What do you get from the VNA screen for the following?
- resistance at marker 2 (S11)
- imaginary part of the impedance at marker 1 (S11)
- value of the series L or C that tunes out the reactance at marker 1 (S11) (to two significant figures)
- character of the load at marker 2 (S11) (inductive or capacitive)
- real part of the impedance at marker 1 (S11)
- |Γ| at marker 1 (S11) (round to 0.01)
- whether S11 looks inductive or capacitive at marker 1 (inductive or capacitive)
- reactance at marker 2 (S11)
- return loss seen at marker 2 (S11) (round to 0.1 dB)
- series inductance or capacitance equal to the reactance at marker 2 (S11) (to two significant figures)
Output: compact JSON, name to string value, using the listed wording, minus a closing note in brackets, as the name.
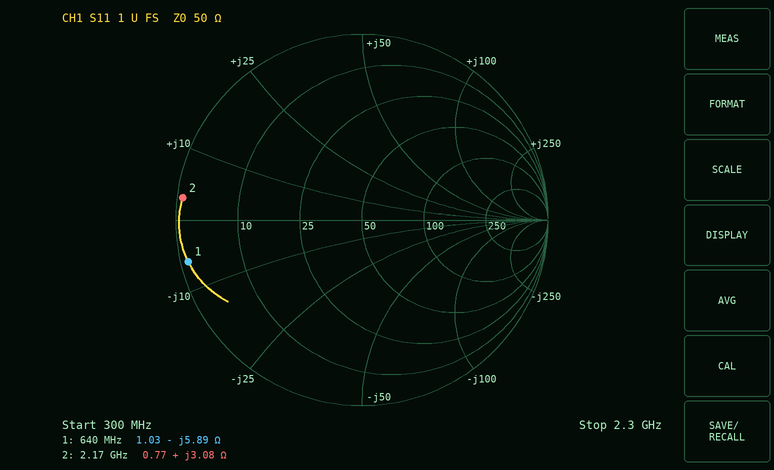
{"resistance at marker 2": "0.77 Ω", "imaginary part of the impedance at marker 1": "-5.89 Ω", "value of the series L or C that tunes out the reactance at marker 1 (S11)": "1.5 nH", "character of the load at marker 2 (S11)": "inductive", "real part of the impedance at marker 1": "1.03 Ω", "|Γ| at marker 1 (S11)": "0.96", "whether S11 looks inductive or capacitive at marker 1": "capacitive", "reactance at marker 2": "+3.08 Ω", "return loss seen at marker 2 (S11)": "0.3 dB", "series inductance or capacitance equal to the reactance at marker 2 (S11)": "230 pH"}
